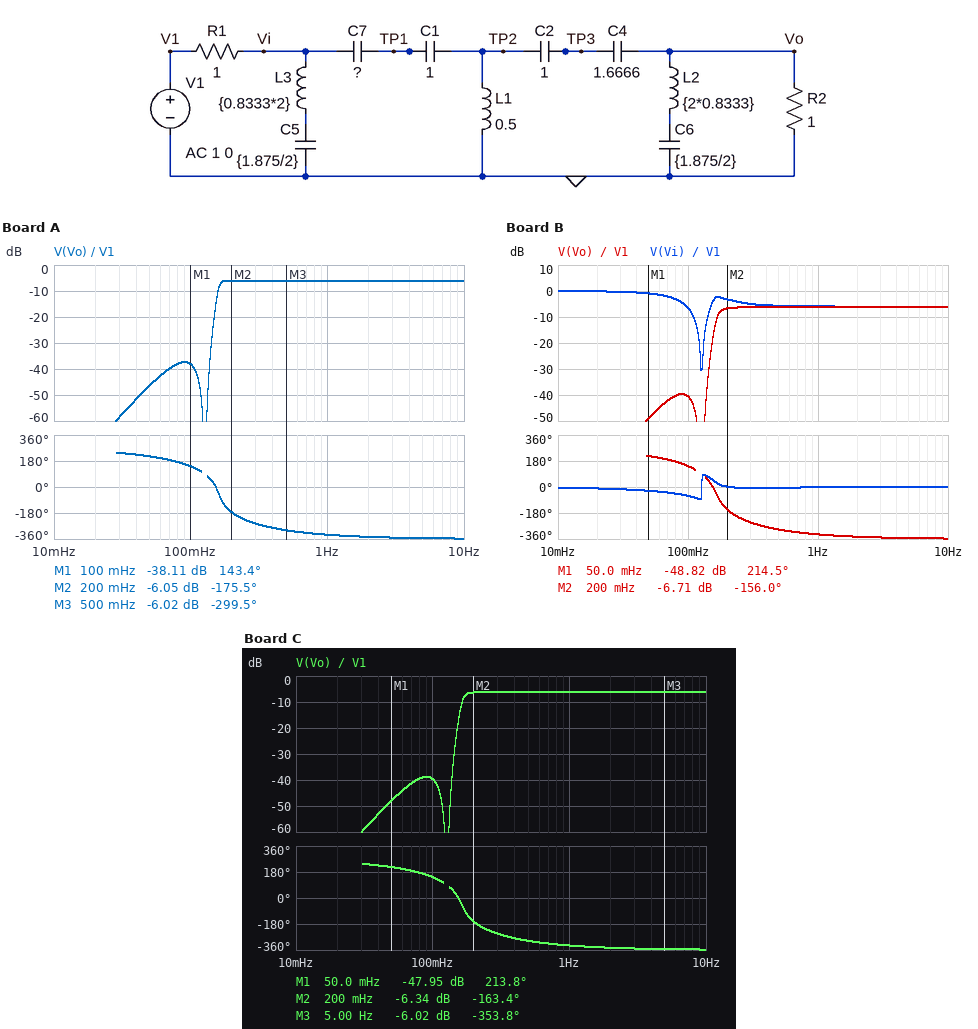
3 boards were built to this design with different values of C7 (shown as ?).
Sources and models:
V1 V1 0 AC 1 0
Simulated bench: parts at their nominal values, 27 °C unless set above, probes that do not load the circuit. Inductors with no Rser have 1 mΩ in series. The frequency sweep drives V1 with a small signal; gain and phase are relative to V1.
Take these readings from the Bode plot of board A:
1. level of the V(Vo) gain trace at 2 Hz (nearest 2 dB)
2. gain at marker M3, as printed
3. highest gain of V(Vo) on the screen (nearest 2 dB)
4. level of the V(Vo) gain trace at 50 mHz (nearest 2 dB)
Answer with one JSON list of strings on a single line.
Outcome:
["-6 dB", "-6.02 dB", "-6 dB", "-46 dB"]
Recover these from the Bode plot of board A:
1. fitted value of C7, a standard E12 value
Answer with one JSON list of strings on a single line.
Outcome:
["1.5 F"]
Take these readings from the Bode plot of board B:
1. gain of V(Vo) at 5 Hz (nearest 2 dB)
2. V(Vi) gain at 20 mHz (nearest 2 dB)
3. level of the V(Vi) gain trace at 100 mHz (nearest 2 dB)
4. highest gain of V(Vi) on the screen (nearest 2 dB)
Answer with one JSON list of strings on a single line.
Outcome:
["-6 dB", "0 dB", "-6 dB", "0 dB"]
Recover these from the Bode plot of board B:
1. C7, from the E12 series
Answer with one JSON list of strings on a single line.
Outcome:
["820 mF"]
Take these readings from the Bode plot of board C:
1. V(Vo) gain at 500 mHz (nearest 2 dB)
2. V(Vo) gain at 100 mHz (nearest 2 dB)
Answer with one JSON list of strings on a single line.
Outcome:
["-6 dB", "-40 dB"]
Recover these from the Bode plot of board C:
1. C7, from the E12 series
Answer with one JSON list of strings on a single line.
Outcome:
["1 F"]
